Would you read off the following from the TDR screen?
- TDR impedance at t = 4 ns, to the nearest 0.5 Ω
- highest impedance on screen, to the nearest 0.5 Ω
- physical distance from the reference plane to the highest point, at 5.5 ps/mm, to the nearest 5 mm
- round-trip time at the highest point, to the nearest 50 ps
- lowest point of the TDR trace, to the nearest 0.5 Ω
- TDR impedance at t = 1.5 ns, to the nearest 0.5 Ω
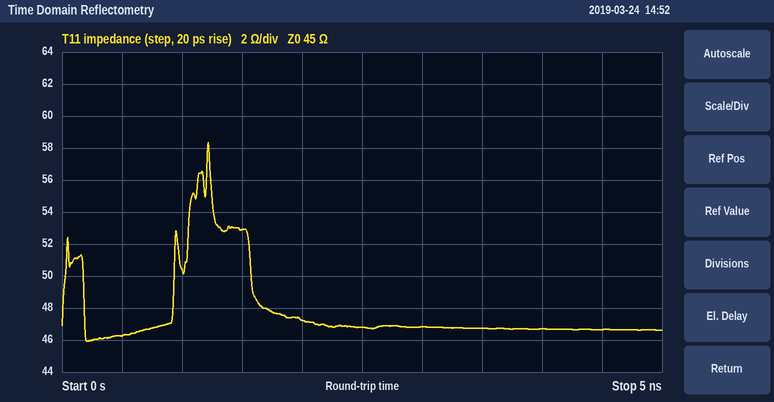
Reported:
46.5 Ω
58.5 Ω
110 mm
1.20 ns
46.0 Ω
53.0 Ω
